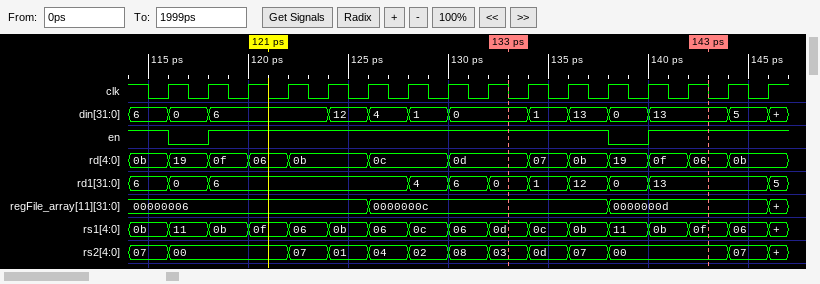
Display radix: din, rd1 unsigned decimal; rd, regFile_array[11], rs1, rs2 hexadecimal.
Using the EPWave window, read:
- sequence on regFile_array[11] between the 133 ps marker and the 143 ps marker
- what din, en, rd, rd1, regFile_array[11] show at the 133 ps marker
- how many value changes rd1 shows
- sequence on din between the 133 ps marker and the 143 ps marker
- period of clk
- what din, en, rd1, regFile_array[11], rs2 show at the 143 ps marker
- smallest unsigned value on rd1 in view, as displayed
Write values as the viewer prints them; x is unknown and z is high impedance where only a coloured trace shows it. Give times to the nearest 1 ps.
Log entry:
0000000c, 0000000d
din=0, en=1, rd=0d, rd1=0, regFile_array[11]=0000000c
10
0, 1, 13, 0, 13
2 ps
din=13, en=1, rd1=13, regFile_array[11]=0000000d, rs2=00
0
